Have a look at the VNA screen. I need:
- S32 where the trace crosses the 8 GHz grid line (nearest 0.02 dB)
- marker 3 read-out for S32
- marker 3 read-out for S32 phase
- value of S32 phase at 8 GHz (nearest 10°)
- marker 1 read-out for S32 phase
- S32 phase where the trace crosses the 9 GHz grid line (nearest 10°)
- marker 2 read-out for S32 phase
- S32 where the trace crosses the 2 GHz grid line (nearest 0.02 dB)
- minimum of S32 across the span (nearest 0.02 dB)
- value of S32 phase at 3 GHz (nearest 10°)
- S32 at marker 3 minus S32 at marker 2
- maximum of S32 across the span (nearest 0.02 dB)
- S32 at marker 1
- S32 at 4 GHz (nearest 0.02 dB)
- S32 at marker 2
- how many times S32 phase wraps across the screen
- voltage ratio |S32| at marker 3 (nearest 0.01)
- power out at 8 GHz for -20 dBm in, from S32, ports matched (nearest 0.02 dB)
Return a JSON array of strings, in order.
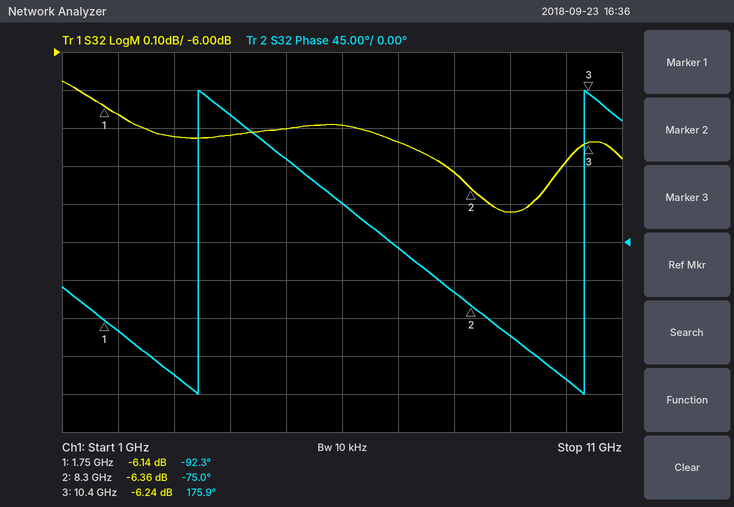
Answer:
["-6.32 dB", "-6.24 dB", "175.9°", "-60°", "-92.3°", "-110°", "-75.0°", "-6.16 dB", "-6.42 dB", "-160°", "0.12 dB", "-6.08 dB", "-6.14 dB", "-6.22 dB", "-6.36 dB", "2", "0.49", "-26.32 dBm"]
